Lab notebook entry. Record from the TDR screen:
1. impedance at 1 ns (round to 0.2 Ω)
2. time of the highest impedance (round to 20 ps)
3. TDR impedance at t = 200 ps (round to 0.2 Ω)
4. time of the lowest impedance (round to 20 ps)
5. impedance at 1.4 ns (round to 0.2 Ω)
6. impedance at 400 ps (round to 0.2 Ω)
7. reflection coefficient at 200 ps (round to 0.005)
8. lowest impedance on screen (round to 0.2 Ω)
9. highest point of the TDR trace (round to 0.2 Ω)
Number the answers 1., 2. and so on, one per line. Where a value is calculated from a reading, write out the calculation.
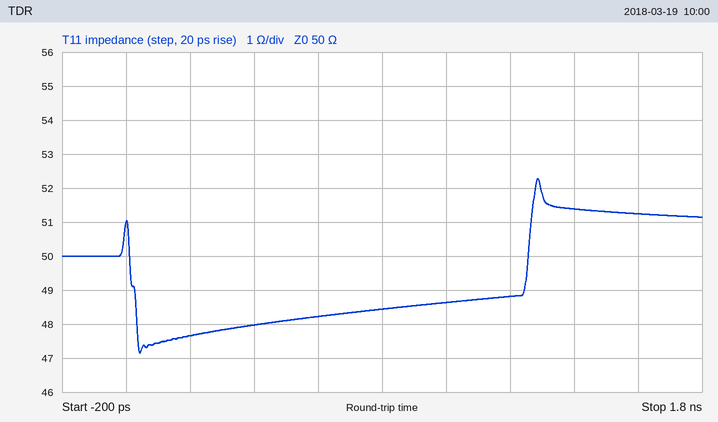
1. 48.6 Ω
2. 1.28 ns
3. 47.6 Ω
4. 40 ps
5. 51.4 Ω
6. 48.0 Ω
7. (47.6 − 50)/(47.6 + 50) ≈ -0.025
8. 47.2 Ω
9. 52.2 Ω
